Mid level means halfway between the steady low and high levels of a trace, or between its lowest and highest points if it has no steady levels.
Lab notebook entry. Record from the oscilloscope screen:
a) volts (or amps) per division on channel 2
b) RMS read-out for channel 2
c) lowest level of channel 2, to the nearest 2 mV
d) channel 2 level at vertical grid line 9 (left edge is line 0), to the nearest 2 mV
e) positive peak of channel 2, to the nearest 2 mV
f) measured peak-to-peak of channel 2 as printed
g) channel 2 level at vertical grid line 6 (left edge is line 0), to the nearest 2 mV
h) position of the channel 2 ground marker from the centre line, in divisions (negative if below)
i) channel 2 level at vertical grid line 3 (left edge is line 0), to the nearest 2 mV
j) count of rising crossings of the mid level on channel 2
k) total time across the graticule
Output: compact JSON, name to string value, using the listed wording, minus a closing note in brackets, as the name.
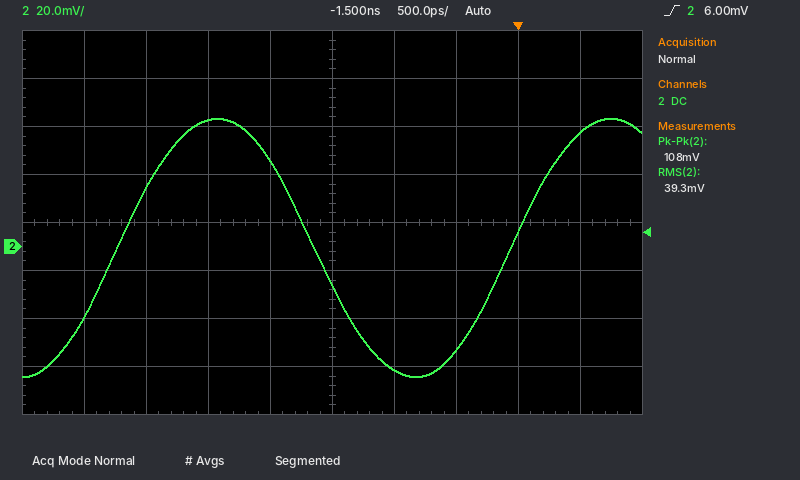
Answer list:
{"volts (or amps) per division on channel 2": "20 mV", "RMS read-out for channel 2": "39.3 mV", "lowest level of channel 2, to the nearest 2 mV": "-54 mV", "channel 2 level at vertical grid line 9 (left edge is line 0), to the nearest 2 mV": "48 mV", "positive peak of channel 2, to the nearest 2 mV": "54 mV", "measured peak-to-peak of channel 2 as printed": "108 mV", "channel 2 level at vertical grid line 6 (left edge is line 0), to the nearest 2 mV": "-52 mV", "position of the channel 2 ground marker from the centre line, in divisions": "-0.5 div", "channel 2 level at vertical grid line 3 (left edge is line 0), to the nearest 2 mV": "52 mV", "count of rising crossings of the mid level on channel 2": "2", "total time across the graticule": "5 ns"}
